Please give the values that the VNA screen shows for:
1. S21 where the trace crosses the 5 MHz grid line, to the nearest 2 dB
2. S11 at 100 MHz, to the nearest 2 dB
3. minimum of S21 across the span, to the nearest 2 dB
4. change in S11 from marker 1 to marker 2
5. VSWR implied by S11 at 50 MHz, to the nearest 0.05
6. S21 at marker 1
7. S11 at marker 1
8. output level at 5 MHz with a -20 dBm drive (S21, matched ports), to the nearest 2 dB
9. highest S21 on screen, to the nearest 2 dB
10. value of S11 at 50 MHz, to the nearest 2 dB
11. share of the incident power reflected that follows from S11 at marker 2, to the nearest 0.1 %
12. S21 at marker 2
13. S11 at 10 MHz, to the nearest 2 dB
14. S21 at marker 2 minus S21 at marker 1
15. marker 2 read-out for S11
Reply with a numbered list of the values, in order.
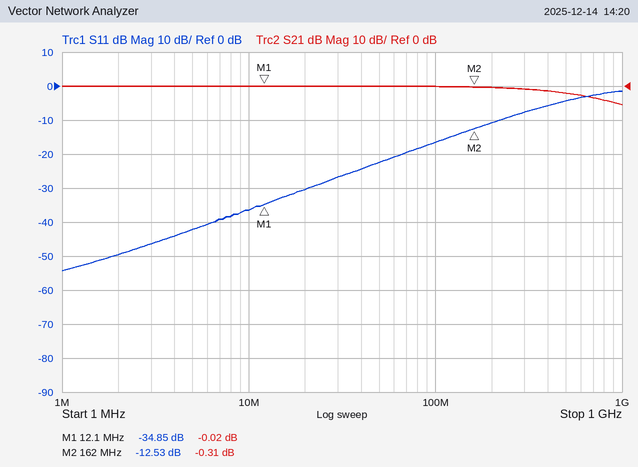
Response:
1. 0 dB
2. -16 dB
3. -6 dB
4. 22.32 dB
5. 1.15
6. -0.02 dB
7. -34.85 dB
8. -20 dBm
9. 0 dB
10. -22 dB
11. 5.6 %
12. -0.31 dB
13. -36 dB
14. -0.29 dB
15. -12.53 dB
